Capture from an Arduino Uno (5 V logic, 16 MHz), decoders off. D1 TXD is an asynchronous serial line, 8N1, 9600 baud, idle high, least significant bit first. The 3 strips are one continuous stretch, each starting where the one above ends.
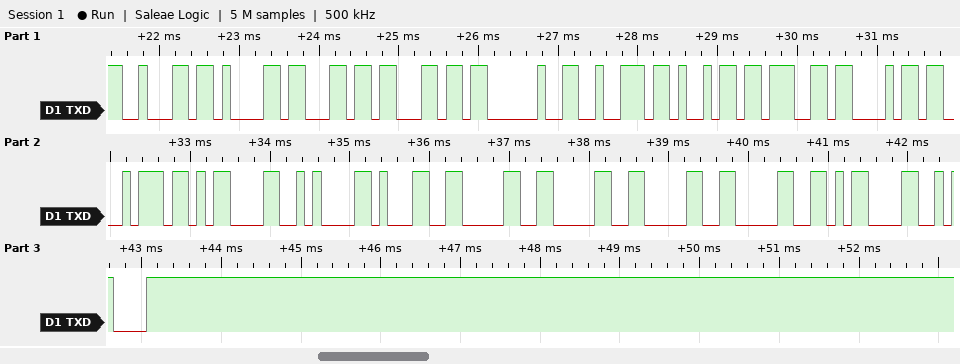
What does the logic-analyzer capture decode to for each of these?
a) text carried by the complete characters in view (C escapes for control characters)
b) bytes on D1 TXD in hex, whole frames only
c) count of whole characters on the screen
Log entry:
"ball right\r\n10000\r\n"
62 61 6C 6C 20 72 69 67 68 74 0D 0A 31 30 30 30 30 0D 0A
19
